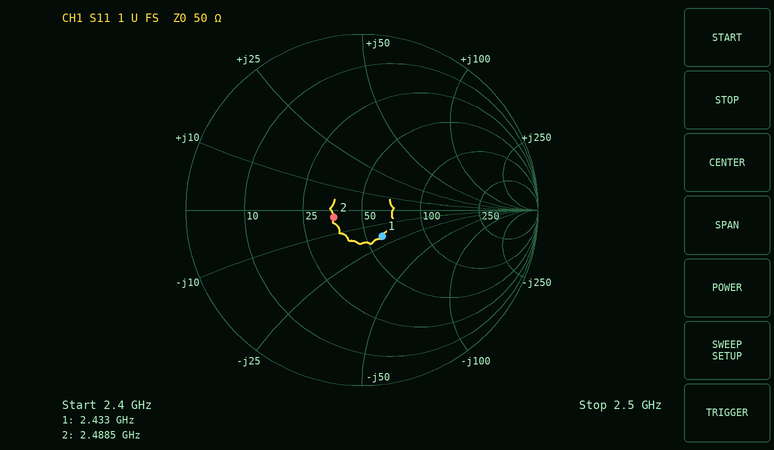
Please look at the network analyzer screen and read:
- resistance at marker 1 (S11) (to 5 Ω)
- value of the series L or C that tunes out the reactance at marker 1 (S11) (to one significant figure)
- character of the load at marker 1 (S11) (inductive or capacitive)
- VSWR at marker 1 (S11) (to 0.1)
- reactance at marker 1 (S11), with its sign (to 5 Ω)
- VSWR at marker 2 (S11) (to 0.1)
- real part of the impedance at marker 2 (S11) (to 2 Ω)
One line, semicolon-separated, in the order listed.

60 Ω; 1 nH; capacitive; 1.5; -20 Ω; 1.4; 36 Ω
